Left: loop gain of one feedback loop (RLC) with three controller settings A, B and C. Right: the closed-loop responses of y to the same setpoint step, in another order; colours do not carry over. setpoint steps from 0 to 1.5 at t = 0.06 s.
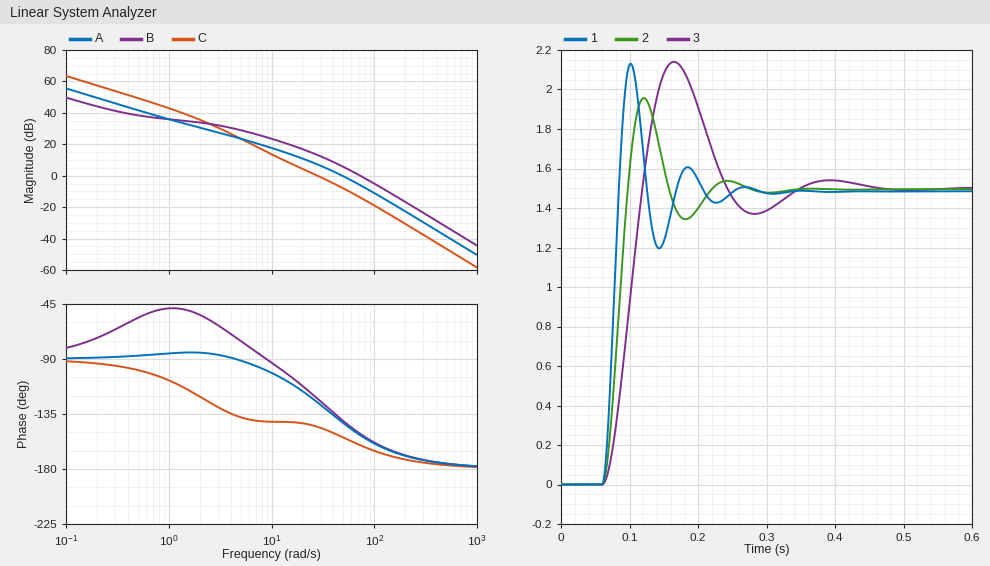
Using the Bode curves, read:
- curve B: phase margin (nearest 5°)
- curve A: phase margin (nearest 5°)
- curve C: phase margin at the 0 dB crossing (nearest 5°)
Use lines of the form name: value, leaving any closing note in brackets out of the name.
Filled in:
curve B: phase margin: 30°
curve A: phase margin: 40°
curve C: phase margin at the 0 dB crossing: 35°
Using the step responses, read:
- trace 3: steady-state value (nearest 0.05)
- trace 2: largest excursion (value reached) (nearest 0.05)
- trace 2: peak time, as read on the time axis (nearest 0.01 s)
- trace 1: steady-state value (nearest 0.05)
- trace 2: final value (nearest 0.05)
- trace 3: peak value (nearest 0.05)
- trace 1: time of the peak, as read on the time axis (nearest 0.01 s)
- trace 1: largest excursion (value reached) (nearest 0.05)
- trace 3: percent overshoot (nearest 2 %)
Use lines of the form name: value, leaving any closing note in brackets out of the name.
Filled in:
trace 3: steady-state value: 1.50
trace 2: largest excursion (value reached): 1.95
trace 2: peak time, as read on the time axis: 0.12 s
trace 1: steady-state value: 1.50
trace 2: final value: 1.50
trace 3: peak value: 2.15
trace 1: time of the peak, as read on the time axis: 0.10 s
trace 1: largest excursion (value reached): 2.15
trace 3: percent overshoot: 42 %
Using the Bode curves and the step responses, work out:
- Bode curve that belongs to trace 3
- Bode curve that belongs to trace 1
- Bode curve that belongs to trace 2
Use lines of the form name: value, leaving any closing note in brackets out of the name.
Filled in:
Bode curve that belongs to trace 3: C
Bode curve that belongs to trace 1: B
Bode curve that belongs to trace 2: A
